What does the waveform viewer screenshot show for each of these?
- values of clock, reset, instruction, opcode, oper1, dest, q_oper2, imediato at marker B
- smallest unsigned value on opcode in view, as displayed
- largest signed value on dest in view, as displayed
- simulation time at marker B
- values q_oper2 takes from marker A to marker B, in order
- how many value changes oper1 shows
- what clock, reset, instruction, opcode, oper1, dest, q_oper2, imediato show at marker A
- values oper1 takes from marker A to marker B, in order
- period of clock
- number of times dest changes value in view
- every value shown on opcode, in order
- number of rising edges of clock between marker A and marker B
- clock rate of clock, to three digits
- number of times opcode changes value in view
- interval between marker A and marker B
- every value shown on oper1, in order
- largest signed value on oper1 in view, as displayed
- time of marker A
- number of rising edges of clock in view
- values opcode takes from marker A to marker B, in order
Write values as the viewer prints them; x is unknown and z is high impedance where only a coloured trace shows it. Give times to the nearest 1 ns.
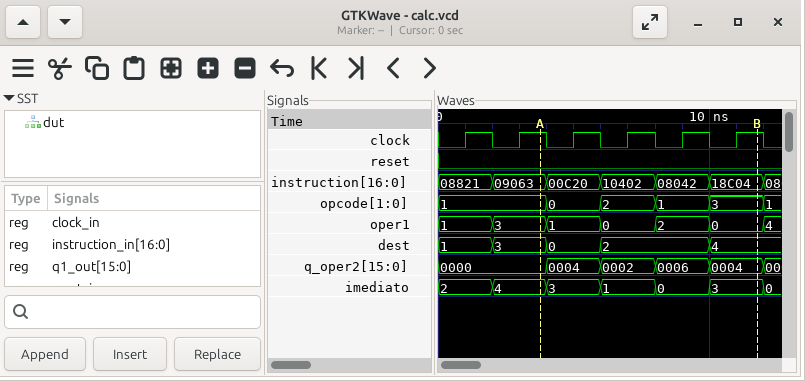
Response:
clock=1, reset=0, instruction=18C04, opcode=3, oper1=0, dest=4, q_oper2=0004, imediato=3
0
4
12 ns
0000, 0004, 0002, 0006, 0004
6
clock=1, reset=0, instruction=09063, opcode=1, oper1=3, dest=3, q_oper2=0000, imediato=4
3, 1, 0, 2, 0
2 ns
4
1, 0, 2, 1, 3, 1
4
500 MHz
5
8 ns
1, 3, 1, 0, 2, 0, 4
4
4 ns
6
1, 0, 2, 1, 3
